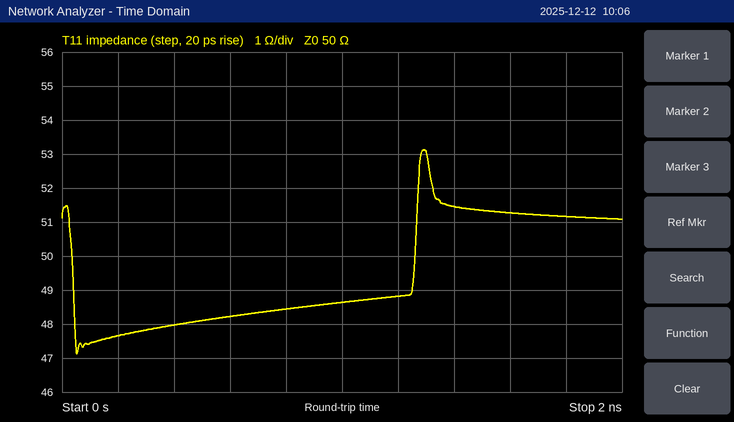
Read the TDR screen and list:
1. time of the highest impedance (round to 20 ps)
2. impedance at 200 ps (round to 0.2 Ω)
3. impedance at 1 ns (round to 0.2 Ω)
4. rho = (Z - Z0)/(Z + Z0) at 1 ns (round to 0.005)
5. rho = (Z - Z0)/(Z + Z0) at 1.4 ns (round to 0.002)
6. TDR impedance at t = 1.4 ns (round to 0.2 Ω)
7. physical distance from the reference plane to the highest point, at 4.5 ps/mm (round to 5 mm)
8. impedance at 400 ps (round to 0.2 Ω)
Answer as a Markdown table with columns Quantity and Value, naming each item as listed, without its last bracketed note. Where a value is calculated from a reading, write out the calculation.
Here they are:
| Quantity | Value |
|---|---|
| time of the highest impedance | 1.30 ns |
| impedance at 200 ps | 47.6 Ω |
| impedance at 1 ns | 48.6 Ω |
| rho = (Z - Z0)/(Z + Z0) at 1 ns | (48.6 − 50)/(48.6 + 50) ≈ -0.0142, so -0.015 to the nearest 0.005 |
| rho = (Z - Z0)/(Z + Z0) at 1.4 ns | (51.4 − 50)/(51.4 + 50) ≈ +0.014 |
| TDR impedance at t = 1.4 ns | 51.4 Ω |
| physical distance from the reference plane to the highest point, at 4.5 ps/mm | 1.30 ns / 2 / 4.5 ps/mm ≈ 144 mm, so 145 mm to the nearest 5 mm |
| impedance at 400 ps | 48.0 Ω |
